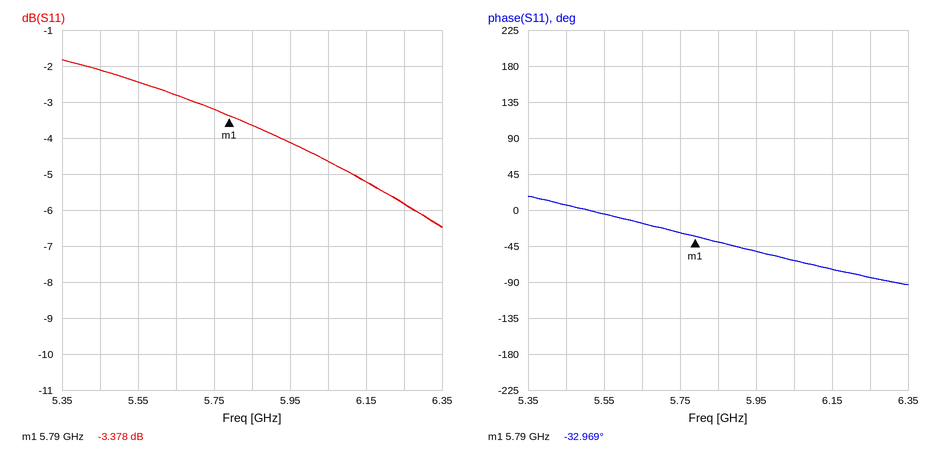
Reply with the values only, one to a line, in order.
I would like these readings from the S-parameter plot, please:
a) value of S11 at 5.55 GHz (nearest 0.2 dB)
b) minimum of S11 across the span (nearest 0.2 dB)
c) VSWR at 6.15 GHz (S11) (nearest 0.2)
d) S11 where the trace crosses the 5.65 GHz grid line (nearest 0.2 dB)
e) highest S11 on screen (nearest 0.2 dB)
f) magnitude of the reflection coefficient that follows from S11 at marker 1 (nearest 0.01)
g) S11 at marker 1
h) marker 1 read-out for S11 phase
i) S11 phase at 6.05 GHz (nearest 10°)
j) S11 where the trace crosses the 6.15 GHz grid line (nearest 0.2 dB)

-2.4 dB
-6.4 dB
3.4
-2.8 dB
-1.8 dB
0.68
-3.378 dB
-32.969°
-60°
-5.2 dB
